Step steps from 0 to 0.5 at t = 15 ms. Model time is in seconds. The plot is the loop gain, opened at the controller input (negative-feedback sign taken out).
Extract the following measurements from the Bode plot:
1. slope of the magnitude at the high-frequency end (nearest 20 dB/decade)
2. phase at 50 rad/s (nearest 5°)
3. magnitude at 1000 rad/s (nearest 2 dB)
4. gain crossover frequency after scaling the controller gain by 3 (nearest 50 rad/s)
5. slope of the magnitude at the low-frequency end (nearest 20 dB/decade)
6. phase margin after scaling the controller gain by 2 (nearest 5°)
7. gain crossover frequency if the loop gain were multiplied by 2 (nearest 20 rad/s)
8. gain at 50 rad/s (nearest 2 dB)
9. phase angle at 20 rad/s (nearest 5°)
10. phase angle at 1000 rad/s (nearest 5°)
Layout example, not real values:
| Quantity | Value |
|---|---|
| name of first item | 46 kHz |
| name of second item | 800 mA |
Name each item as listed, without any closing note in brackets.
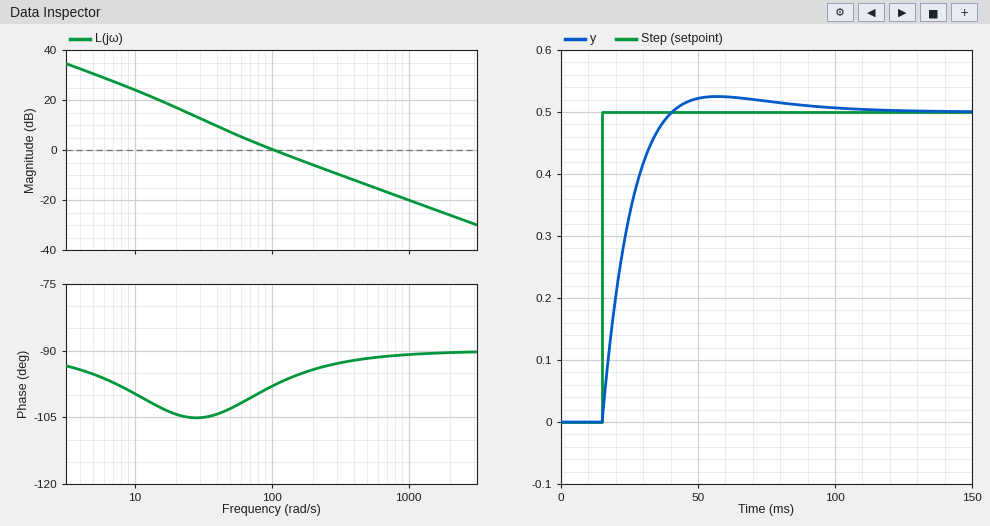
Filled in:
| Quantity | Value |
|---|---|
| slope of the magnitude at the high-frequency end | -20 dB/decade |
| phase at 50 rad/s | -105° |
| magnitude at 1000 rad/s | -20 dB |
| gain crossover frequency after scaling the controller gain by 3 | 300 rad/s |
| slope of the magnitude at the low-frequency end | -20 dB/decade |
| phase margin after scaling the controller gain by 2 | 85° |
| gain crossover frequency if the loop gain were multiplied by 2 | 200 rad/s |
| gain at 50 rad/s | 8 dB |
| phase angle at 20 rad/s | -105° |
| phase angle at 1000 rad/s | -90° |
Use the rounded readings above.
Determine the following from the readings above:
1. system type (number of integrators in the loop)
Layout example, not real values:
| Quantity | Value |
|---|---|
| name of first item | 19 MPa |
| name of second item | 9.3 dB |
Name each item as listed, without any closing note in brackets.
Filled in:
| Quantity | Value |
|---|---|
| system type | 1 |
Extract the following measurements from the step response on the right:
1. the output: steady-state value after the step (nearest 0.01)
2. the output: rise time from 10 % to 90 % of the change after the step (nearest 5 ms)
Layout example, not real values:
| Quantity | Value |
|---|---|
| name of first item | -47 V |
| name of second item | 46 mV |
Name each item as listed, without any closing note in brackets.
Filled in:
| Quantity | Value |
|---|---|
| the output: steady-state value after the step | 0.50 |
| the output: rise time from 10 % to 90 % of the change after the step | 15 ms |
